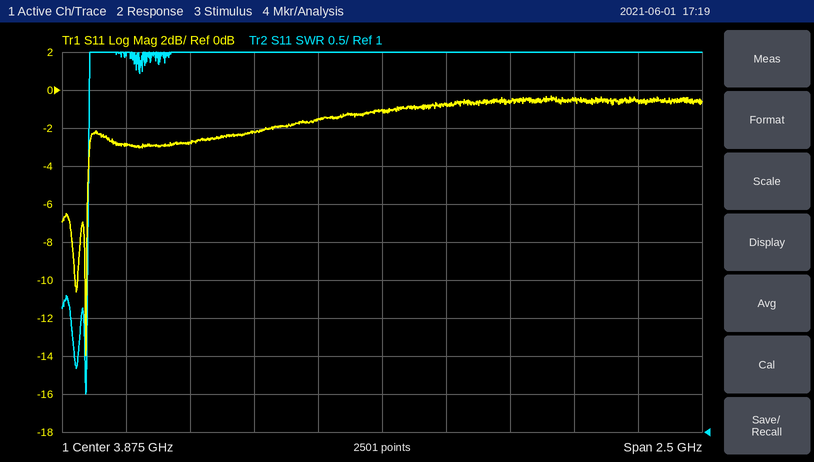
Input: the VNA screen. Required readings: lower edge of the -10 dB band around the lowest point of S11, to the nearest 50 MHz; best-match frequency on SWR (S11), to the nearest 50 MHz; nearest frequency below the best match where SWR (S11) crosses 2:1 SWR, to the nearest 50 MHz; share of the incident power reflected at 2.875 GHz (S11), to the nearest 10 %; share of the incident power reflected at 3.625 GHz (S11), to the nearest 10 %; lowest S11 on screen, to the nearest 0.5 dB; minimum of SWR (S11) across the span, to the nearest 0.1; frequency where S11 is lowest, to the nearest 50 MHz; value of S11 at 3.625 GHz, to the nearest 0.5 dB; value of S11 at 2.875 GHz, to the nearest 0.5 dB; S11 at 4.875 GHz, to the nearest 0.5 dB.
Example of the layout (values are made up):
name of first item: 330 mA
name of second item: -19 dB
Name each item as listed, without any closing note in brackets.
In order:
lower edge of the -10 dB band around the lowest point of S11, to the nearest 50 MHz: 2.70 GHz
best-match frequency on SWR (S11), to the nearest 50 MHz: 2.70 GHz
nearest frequency below the best match where SWR (S11) crosses 2:1 SWR, to the nearest 50 MHz: 2.70 GHz
share of the incident power reflected at 2.875 GHz (S11), to the nearest 10 %: 50 %
share of the incident power reflected at 3.625 GHz (S11), to the nearest 10 %: 70 %
lowest S11 on screen, to the nearest 0.5 dB: -14.0 dB
minimum of SWR (S11) across the span, to the nearest 0.1: 1.5
frequency where S11 is lowest, to the nearest 50 MHz: 2.70 GHz
value of S11 at 3.625 GHz, to the nearest 0.5 dB: -1.5 dB
value of S11 at 2.875 GHz, to the nearest 0.5 dB: -3.0 dB
S11 at 4.875 GHz, to the nearest 0.5 dB: -0.5 dB
